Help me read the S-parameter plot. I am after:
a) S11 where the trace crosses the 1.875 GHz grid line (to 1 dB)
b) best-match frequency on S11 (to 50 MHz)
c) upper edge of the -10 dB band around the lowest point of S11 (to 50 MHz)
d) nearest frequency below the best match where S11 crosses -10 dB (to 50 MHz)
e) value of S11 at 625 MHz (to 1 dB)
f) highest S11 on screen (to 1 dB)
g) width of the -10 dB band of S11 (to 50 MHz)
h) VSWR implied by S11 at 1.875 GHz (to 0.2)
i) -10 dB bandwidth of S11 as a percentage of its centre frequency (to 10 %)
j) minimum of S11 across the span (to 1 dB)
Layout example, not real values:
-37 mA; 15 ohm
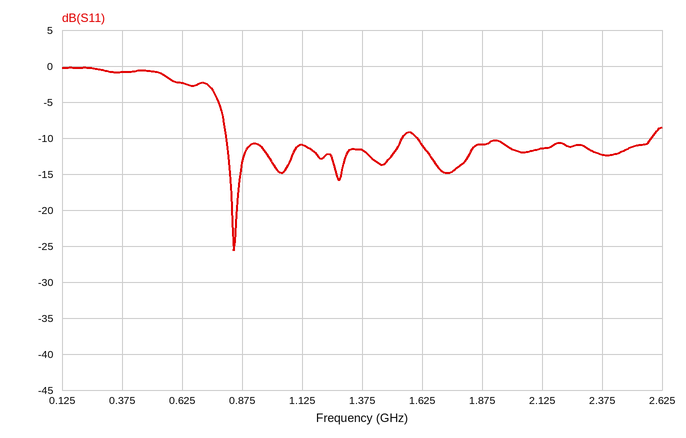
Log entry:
-11 dB; 850 MHz; 1.55 GHz; 800 MHz; -2 dB; 0 dB; 750 MHz; 1.8; 60 %; -26 dB
